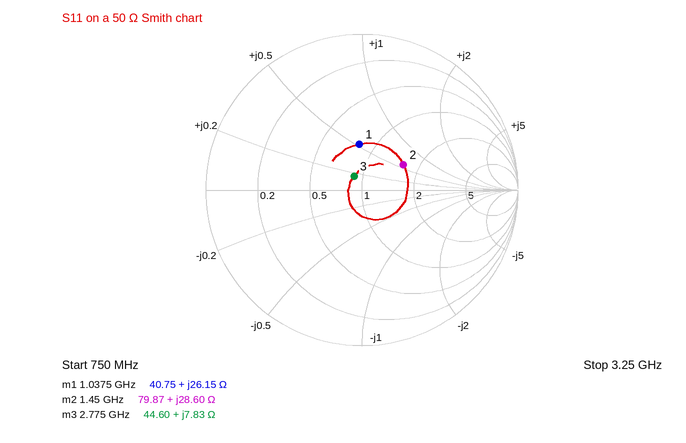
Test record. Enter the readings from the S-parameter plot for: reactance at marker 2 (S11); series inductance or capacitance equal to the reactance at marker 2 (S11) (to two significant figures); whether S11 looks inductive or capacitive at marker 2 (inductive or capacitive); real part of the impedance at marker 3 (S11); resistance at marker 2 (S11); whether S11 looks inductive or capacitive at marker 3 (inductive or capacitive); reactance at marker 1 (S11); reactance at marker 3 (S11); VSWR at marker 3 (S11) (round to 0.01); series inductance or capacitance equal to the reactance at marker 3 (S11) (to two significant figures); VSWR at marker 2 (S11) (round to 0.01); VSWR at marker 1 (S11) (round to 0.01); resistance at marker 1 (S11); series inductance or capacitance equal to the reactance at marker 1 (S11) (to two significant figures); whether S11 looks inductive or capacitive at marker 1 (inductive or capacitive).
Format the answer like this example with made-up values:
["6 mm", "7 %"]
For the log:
["+28.60 Ω", "3.1 nH", "inductive", "44.60 Ω", "79.87 Ω", "inductive", "+26.15 Ω", "+7.83 Ω", "1.22", "450 pH", "1.90", "1.83", "40.75 Ω", "4.0 nH", "inductive"]
